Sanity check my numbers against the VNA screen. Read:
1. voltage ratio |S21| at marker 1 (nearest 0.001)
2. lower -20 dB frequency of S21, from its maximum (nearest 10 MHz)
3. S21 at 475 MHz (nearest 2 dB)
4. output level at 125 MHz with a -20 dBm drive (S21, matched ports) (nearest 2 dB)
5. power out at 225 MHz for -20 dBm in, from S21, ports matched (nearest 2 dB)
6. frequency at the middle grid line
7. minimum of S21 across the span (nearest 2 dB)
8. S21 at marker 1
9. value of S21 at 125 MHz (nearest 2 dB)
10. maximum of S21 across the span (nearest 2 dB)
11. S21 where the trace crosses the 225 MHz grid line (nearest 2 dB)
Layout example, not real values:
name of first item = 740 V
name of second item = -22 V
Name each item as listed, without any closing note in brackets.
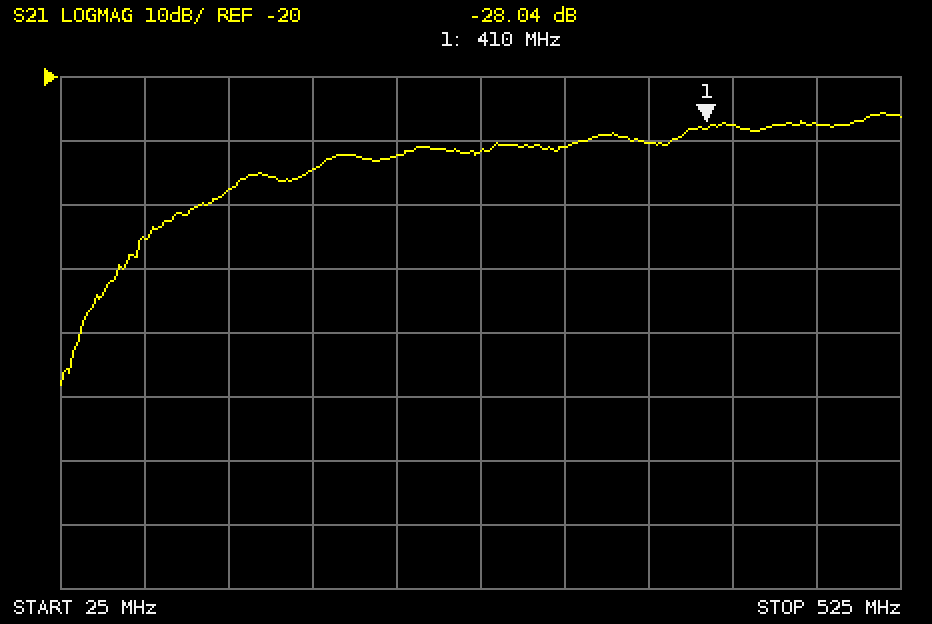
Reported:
voltage ratio |S21| at marker 1 = 0.040
lower -20 dB frequency of S21, from its maximum = 70 MHz
S21 at 475 MHz = -28 dB
output level at 125 MHz with a -20 dBm drive (S21, matched ports) = -58 dBm
power out at 225 MHz for -20 dBm in, from S21, ports matched = -52 dBm
frequency at the middle grid line = 275 MHz
minimum of S21 across the span = -68 dB
S21 at marker 1 = -28.04 dB
value of S21 at 125 MHz = -38 dB
maximum of S21 across the span = -26 dB
S21 where the trace crosses the 225 MHz grid line = -32 dB
